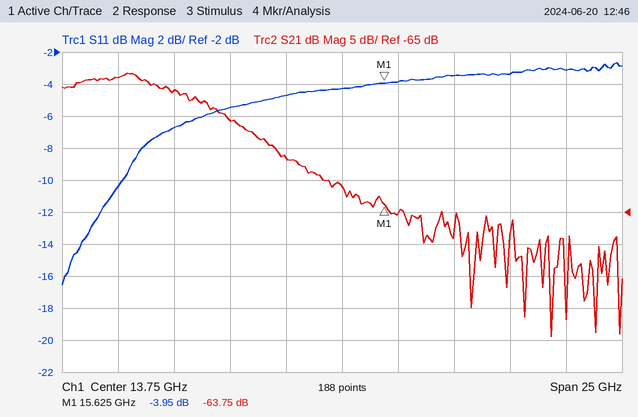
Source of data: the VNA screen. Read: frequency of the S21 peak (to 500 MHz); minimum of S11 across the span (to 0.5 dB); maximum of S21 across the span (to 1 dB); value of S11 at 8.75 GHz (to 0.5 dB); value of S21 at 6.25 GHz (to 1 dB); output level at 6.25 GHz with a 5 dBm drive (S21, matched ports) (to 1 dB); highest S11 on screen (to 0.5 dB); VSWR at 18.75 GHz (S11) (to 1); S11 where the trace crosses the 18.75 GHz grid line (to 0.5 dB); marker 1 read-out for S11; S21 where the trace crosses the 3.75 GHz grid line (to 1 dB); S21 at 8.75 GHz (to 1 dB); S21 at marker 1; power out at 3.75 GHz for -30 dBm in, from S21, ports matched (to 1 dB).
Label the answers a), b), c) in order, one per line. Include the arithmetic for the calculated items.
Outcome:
a) 4.0 GHz
b) -16.5 dB
c) -43 dB
d) -5.5 dB
e) -46 dB
f) 5 dBm + (-46 dB) = -41 dBm
g) -2.5 dB
h) |Γ| = 10^(-3.5/20) = 0.6683; VSWR = (1 + 0.6683)/(1 − 0.6683) ≈ 5
i) -3.5 dB
j) -3.95 dB
k) -44 dB
l) -51 dB
m) -63.75 dB
n) -30 dBm + (-44 dB) = -74 dBm
